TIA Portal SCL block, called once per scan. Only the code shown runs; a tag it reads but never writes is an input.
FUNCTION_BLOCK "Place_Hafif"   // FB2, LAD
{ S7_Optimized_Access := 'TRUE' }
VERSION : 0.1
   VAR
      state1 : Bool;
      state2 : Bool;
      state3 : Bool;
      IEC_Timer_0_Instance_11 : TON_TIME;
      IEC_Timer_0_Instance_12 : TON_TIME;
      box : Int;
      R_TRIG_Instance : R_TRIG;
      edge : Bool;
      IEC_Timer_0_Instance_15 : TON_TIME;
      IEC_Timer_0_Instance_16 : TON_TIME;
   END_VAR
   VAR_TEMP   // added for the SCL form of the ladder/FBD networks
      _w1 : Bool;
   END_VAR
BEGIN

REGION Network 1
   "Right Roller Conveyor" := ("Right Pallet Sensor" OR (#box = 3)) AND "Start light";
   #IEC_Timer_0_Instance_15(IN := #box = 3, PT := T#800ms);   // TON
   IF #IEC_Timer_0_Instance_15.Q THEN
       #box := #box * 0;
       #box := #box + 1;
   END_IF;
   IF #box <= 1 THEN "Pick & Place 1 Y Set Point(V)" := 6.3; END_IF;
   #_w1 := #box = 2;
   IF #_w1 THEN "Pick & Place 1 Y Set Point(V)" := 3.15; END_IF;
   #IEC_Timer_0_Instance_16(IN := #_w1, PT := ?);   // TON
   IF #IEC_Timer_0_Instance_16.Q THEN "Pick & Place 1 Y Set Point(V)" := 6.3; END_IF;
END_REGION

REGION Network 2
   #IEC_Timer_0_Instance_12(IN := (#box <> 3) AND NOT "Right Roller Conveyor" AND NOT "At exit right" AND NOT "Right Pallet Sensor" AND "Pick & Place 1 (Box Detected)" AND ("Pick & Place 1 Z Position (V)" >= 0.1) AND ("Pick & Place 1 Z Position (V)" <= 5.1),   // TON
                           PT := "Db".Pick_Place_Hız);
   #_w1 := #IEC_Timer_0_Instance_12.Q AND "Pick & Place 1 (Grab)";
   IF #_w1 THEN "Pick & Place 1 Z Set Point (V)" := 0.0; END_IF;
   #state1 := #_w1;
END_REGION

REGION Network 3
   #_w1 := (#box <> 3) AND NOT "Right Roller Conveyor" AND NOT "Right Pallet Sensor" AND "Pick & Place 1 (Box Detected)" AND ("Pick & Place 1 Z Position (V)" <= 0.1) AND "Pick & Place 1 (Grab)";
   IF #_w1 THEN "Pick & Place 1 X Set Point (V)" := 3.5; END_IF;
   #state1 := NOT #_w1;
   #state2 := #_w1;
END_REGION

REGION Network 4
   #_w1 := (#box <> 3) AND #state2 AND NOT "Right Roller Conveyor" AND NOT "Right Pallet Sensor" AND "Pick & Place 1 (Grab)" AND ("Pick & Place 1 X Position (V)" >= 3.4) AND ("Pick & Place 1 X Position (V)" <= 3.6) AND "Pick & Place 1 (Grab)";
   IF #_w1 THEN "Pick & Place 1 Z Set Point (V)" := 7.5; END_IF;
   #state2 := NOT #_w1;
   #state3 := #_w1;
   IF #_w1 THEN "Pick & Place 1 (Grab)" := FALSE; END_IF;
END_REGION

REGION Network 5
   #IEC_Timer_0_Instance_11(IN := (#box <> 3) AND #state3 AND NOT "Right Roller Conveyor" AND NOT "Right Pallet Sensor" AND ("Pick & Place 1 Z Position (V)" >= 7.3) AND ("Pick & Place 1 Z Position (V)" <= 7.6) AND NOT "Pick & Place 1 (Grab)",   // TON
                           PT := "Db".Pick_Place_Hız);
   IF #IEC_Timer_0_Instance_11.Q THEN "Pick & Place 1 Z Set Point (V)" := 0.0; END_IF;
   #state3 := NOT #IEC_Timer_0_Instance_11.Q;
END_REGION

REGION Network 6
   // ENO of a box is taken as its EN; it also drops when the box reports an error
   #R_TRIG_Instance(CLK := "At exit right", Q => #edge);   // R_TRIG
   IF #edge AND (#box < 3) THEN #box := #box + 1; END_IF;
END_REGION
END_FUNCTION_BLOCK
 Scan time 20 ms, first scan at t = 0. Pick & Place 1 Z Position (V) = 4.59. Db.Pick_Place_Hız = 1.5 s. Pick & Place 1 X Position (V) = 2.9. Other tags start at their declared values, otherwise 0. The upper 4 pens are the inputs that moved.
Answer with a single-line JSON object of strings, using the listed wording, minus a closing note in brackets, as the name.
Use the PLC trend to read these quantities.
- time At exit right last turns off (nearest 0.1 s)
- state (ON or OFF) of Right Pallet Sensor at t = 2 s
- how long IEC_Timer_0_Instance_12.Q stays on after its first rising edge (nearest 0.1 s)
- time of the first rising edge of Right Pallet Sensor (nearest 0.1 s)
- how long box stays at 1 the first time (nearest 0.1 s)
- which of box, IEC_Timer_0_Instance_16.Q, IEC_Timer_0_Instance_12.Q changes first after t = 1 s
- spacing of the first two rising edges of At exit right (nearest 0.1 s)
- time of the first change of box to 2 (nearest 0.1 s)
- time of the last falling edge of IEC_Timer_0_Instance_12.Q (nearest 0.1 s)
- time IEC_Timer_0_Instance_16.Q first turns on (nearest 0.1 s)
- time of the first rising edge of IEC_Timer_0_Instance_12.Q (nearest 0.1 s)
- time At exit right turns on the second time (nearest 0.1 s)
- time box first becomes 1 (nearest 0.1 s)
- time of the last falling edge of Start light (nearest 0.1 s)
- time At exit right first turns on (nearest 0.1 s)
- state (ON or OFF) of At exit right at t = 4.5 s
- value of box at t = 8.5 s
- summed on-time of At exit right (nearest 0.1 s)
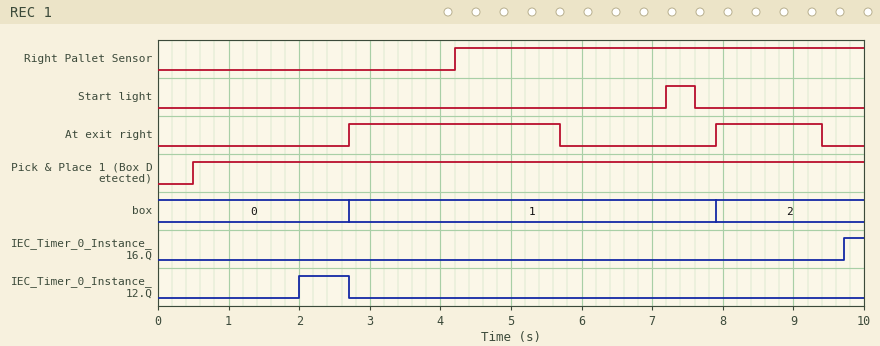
{"time At exit right last turns off": "9.4 s", "state (ON or OFF) of Right Pallet Sensor at t = 2 s": "OFF", "how long IEC_Timer_0_Instance_12.Q stays on after its first rising edge": "0.7 s", "time of the first rising edge of Right Pallet Sensor": "4.2 s", "how long box stays at 1 the first time": "5.2 s", "which of box, IEC_Timer_0_Instance_16.Q, IEC_Timer_0_Instance_12.Q changes first after t = 1 s": "IEC_Timer_0_Instance_12.Q", "spacing of the first two rising edges of At exit right": "5.2 s", "time of the first change of box to 2": "7.9 s", "time of the last falling edge of IEC_Timer_0_Instance_12.Q": "2.7 s", "time IEC_Timer_0_Instance_16.Q first turns on": "9.7 s", "time of the first rising edge of IEC_Timer_0_Instance_12.Q": "2.0 s", "time At exit right turns on the second time": "7.9 s", "time box first becomes 1": "2.7 s", "time of the last falling edge of Start light": "7.6 s", "time At exit right first turns on": "2.7 s", "state (ON or OFF) of At exit right at t = 4.5 s": "ON", "value of box at t = 8.5 s": "2", "summed on-time of At exit right": "4.5 s"}
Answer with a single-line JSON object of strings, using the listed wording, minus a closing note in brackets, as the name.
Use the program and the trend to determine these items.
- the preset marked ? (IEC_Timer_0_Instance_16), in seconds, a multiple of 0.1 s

{"the preset marked ? (IEC_Timer_0_Instance_16), in seconds, a multiple of 0.1 s": "1.8 s"}
